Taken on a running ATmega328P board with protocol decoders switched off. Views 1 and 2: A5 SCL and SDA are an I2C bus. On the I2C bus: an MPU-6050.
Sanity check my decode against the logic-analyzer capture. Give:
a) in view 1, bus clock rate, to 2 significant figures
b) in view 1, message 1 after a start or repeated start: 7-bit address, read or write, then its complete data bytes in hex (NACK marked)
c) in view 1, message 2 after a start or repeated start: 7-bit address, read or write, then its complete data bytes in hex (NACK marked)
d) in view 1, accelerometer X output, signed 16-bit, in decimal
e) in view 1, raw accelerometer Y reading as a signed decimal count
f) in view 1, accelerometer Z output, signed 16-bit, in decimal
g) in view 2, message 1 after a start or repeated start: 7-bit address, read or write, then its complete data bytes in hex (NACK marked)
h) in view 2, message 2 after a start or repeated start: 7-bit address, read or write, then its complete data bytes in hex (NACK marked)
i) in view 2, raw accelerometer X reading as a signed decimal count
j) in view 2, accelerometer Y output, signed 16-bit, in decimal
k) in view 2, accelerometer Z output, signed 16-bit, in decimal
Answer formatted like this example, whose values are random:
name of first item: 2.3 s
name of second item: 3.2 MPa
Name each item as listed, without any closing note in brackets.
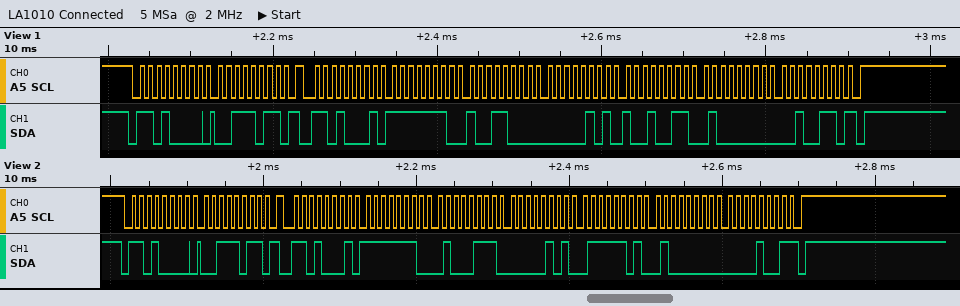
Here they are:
in view 1, bus clock rate, to 2 significant figures: 100 kHz
in view 1, message 1 after a start or repeated start: 7-bit address, read or write, then its complete data bytes in hex: 0x68 write: 3B
in view 1, message 2 after a start or repeated start: 7-bit address, read or write, then its complete data bytes in hex: 0x68 read: FE 98 05 93 40 26 NACK
in view 1, accelerometer X output, signed 16-bit, in decimal: -360
in view 1, raw accelerometer Y reading as a signed decimal count: 1427
in view 1, accelerometer Z output, signed 16-bit, in decimal: 16422
in view 2, message 1 after a start or repeated start: 7-bit address, read or write, then its complete data bytes in hex: 0x68 write: 3B
in view 2, message 2 after a start or repeated start: 7-bit address, read or write, then its complete data bytes in hex: 0x68 read: FE 47 05 7D 40 09 NACK
in view 2, raw accelerometer X reading as a signed decimal count: -441
in view 2, accelerometer Y output, signed 16-bit, in decimal: 1405
in view 2, accelerometer Z output, signed 16-bit, in decimal: 16393
